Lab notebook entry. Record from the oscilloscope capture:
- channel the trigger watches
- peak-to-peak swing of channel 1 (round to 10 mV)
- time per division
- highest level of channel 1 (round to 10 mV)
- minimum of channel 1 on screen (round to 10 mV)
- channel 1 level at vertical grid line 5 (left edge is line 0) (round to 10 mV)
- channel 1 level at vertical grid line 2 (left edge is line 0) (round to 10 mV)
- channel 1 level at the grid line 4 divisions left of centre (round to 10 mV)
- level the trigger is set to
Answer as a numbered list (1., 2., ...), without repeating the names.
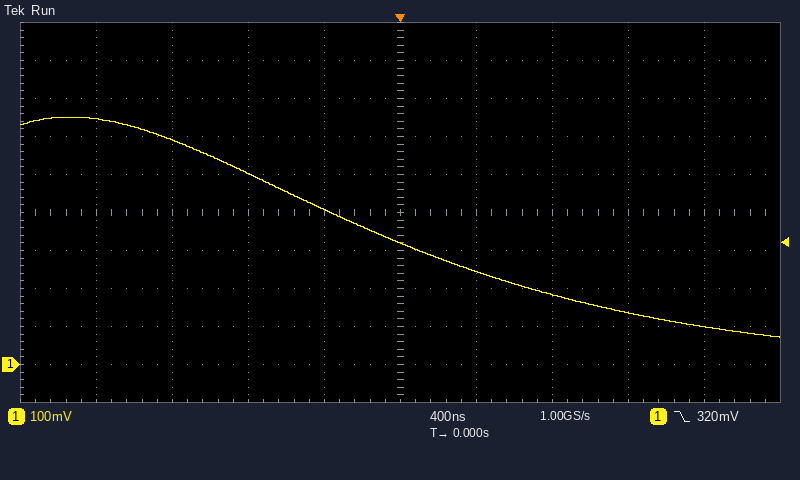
1. channel 1
2. 580 mV
3. 400 ns
4. 650 mV
5. 70 mV
6. 320 mV
7. 590 mV
8. 650 mV
9. 320 mV
